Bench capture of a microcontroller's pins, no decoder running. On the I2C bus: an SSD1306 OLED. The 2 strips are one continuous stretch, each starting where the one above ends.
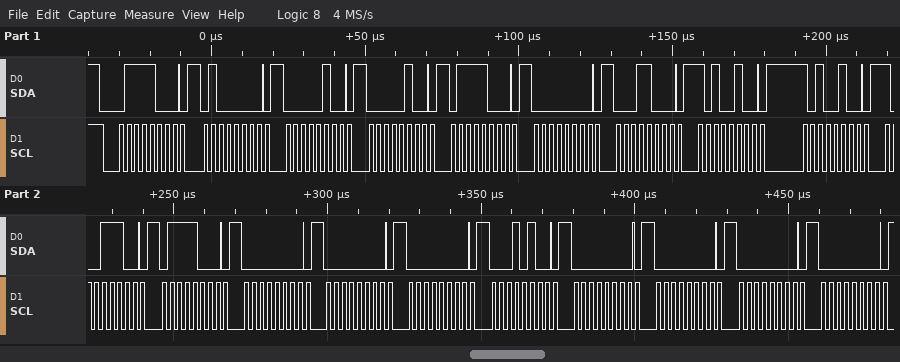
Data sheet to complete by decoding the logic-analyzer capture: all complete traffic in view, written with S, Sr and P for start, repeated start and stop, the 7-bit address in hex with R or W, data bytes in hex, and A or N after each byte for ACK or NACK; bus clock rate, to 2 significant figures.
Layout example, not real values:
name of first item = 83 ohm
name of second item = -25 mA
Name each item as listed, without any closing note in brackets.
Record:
all complete traffic in view, written with S, Sr and P for start, repeated start and stop, the 7-bit address in hex with R or W, data bytes in hex, and A or N after each byte for ACK or NACK = S 3CW A 40 A 04 A 04 A 78 A 00 A 18 A A4 A A4 A 9C A 78 A 00 A 00 A 00 A 14 A 00 A 00 A 00 A 00 A
bus clock rate, to 2 significant figures = 400 kHz
